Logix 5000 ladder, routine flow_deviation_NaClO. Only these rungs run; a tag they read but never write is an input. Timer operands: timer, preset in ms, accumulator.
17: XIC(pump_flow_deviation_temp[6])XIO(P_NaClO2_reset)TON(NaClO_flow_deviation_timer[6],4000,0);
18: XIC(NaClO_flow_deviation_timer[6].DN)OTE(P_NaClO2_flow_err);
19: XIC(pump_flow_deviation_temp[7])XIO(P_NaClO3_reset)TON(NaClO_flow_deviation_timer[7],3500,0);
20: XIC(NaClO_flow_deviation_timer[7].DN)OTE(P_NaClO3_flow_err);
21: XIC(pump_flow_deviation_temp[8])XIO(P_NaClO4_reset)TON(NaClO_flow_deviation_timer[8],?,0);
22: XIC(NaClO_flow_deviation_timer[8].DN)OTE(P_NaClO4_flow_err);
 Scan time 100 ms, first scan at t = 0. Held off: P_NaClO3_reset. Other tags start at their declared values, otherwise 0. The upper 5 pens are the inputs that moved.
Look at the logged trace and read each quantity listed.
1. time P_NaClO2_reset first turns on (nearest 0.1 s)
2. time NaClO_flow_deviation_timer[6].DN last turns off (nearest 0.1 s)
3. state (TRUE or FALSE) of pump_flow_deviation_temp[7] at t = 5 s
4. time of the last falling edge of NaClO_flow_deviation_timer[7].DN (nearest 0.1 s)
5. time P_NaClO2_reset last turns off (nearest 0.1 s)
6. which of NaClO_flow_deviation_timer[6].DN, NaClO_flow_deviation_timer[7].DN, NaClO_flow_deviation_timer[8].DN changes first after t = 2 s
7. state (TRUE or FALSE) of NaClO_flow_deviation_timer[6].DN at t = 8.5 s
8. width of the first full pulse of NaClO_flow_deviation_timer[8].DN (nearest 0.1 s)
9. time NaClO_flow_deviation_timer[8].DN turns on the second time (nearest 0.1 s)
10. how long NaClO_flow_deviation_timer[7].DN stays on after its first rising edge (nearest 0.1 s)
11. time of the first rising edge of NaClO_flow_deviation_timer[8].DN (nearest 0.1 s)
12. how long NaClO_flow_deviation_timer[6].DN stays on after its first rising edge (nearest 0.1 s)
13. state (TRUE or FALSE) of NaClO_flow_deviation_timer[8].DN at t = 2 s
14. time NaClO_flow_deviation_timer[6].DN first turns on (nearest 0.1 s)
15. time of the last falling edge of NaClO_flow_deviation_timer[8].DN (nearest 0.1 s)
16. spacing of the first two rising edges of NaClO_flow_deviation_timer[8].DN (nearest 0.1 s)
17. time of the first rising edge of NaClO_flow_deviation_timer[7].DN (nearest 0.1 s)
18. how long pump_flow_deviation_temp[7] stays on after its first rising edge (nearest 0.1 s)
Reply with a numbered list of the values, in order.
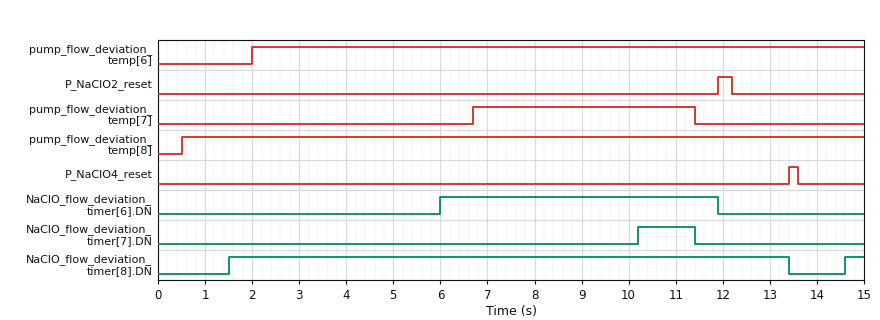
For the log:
1. 11.9 s
2. 11.9 s
3. FALSE
4. 11.4 s
5. 12.2 s
6. NaClO_flow_deviation_timer[6].DN
7. TRUE
8. 11.9 s
9. 14.6 s
10. 1.2 s
11. 1.5 s
12. 5.9 s
13. TRUE
14. 6.0 s
15. 13.4 s
16. 13.1 s
17. 10.2 s
18. 4.7 s
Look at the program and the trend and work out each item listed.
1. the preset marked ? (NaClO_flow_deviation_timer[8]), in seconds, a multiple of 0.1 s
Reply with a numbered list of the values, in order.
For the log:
1. 1.0 s
